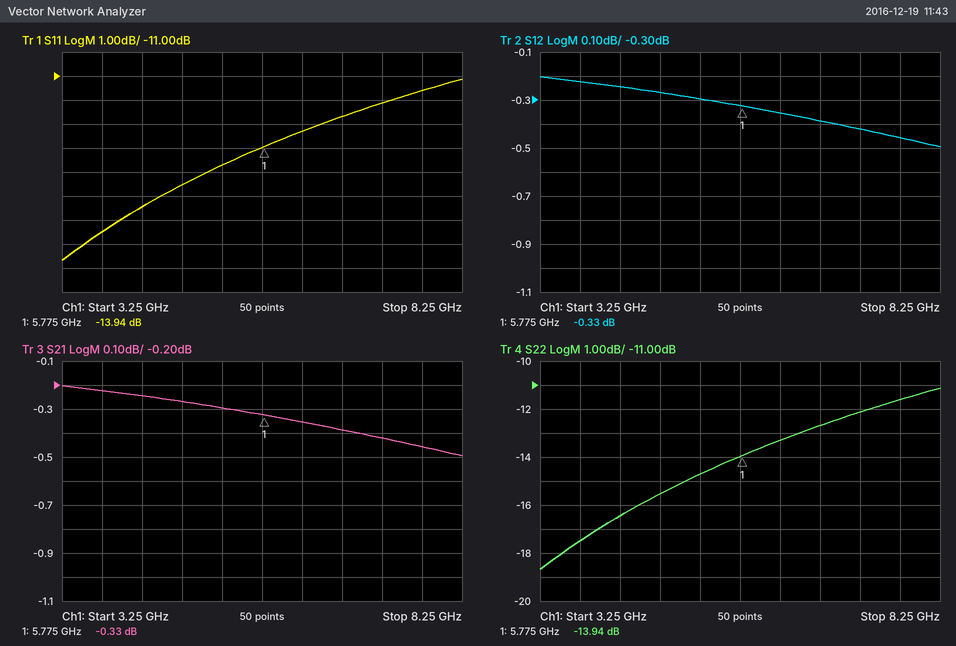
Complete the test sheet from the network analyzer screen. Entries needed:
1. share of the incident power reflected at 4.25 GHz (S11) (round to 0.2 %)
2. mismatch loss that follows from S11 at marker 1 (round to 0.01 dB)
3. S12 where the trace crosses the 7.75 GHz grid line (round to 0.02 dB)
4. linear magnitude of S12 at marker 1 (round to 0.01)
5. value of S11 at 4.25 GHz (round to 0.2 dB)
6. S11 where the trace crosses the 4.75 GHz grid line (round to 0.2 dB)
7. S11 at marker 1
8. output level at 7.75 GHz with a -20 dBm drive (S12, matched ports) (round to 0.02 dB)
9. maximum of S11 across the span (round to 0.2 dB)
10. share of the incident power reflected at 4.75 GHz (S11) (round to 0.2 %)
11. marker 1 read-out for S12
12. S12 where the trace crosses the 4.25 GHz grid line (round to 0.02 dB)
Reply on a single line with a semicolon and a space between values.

2.2 %; 0.18 dB; -0.46 dB; 0.96; -16.4 dB; -15.6 dB; -13.94 dB; -20.46 dBm; -11.2 dB; 2.8 %; -0.33 dB; -0.24 dB
